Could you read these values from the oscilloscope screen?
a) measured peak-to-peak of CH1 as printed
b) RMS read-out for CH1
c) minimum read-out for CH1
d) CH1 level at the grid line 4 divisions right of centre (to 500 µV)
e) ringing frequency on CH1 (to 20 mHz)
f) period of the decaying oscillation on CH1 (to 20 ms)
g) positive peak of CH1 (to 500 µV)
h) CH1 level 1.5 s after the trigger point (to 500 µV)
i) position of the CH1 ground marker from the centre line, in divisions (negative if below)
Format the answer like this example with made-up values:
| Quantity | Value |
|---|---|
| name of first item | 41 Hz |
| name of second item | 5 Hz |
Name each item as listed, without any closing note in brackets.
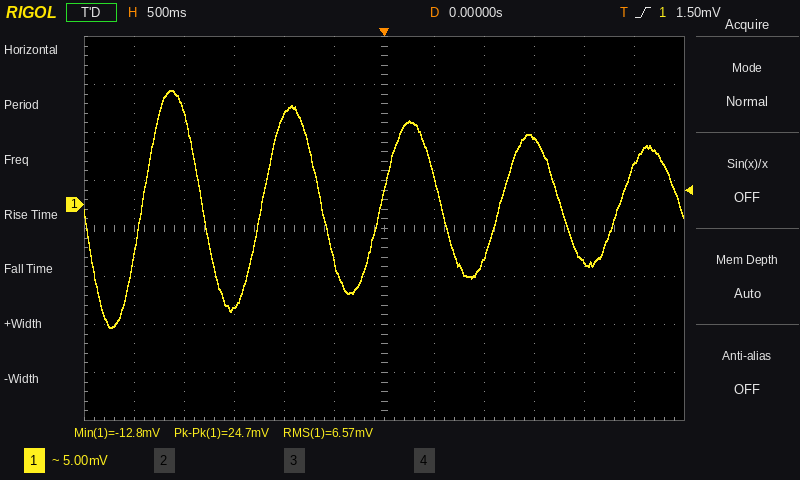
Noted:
| Quantity | Value |
|---|---|
| measured peak-to-peak of CH1 as printed | 24.7 mV |
| RMS read-out for CH1 | 6.57 mV |
| minimum read-out for CH1 | -12.8 mV |
| CH1 level at the grid line 4 divisions right of centre | -6.0 mV |
| ringing frequency on CH1 | 840 mHz |
| period of the decaying oscillation on CH1 | 1.18 s |
| positive peak of CH1 | 12.0 mV |
| CH1 level 1.5 s after the trigger point | 7.0 mV |
| position of the CH1 ground marker from the centre line, in divisions | +0.5 div |
